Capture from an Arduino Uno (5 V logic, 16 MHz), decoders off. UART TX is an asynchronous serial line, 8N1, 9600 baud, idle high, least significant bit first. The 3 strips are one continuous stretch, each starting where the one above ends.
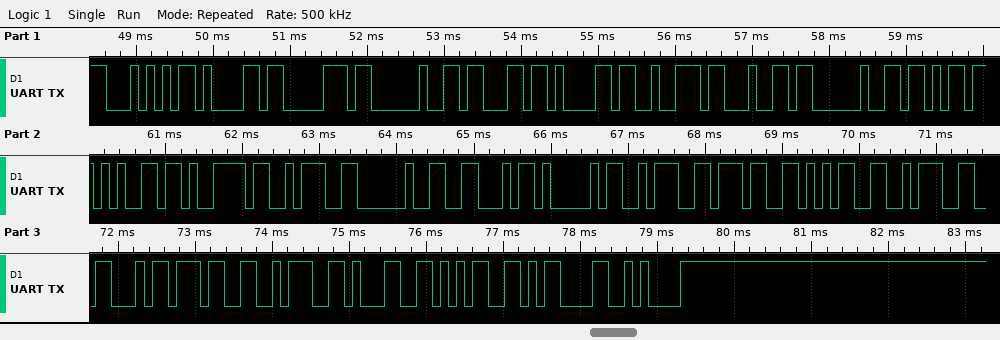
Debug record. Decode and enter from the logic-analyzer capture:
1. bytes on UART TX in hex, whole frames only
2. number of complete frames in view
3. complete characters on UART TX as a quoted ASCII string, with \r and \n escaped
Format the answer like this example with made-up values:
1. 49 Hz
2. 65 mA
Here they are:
1. 54 61 70 20 63 61 72 64 20 6B 65 79 3A 20 46 41 3A 37 35 3A 46 37 3A 31 35 0D 0A
2. 27
3. "Tap card key: FA:75:F7:15\r\n"
